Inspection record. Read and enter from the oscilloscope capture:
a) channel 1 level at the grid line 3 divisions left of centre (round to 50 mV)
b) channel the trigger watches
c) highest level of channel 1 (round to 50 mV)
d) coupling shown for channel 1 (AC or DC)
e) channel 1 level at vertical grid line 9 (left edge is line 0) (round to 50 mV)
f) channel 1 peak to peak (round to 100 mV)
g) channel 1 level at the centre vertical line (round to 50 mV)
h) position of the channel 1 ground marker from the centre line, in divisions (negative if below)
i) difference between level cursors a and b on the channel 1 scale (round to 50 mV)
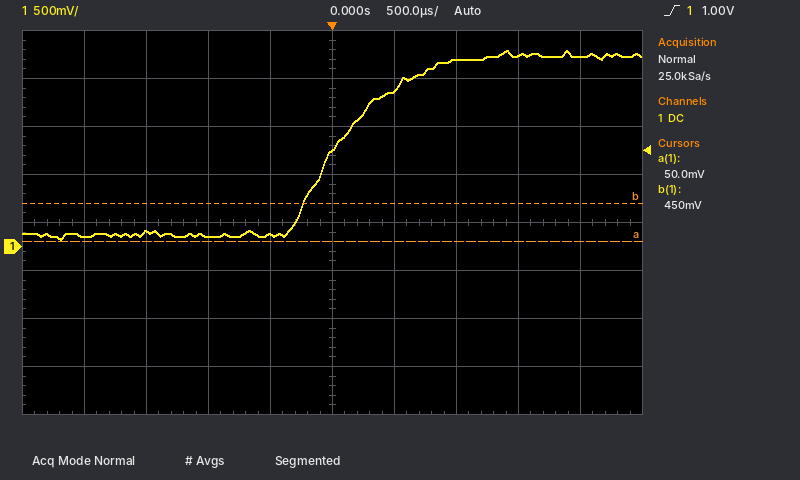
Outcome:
150 mV
channel 1
2.05 V
DC
2.00 V
2.00 V
1.00 V
-0.5 div
400 mV
